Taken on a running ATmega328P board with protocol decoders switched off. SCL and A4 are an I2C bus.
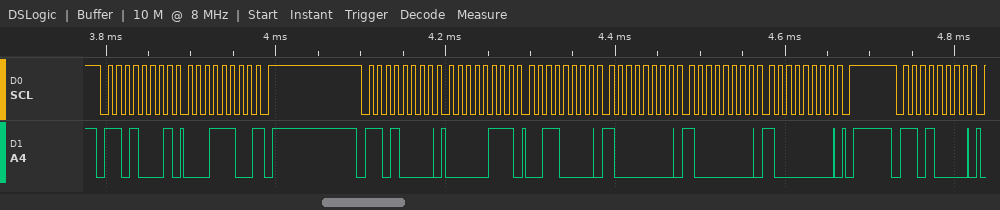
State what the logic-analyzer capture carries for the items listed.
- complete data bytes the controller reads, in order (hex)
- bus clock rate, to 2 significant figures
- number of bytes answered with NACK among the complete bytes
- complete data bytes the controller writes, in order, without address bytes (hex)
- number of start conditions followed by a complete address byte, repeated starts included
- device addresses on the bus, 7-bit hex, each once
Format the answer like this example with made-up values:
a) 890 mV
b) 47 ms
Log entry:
a) 1C
b) 100 kHz
c) 1
d) 07 30 80 80 80
e) 3
f) 0x68
